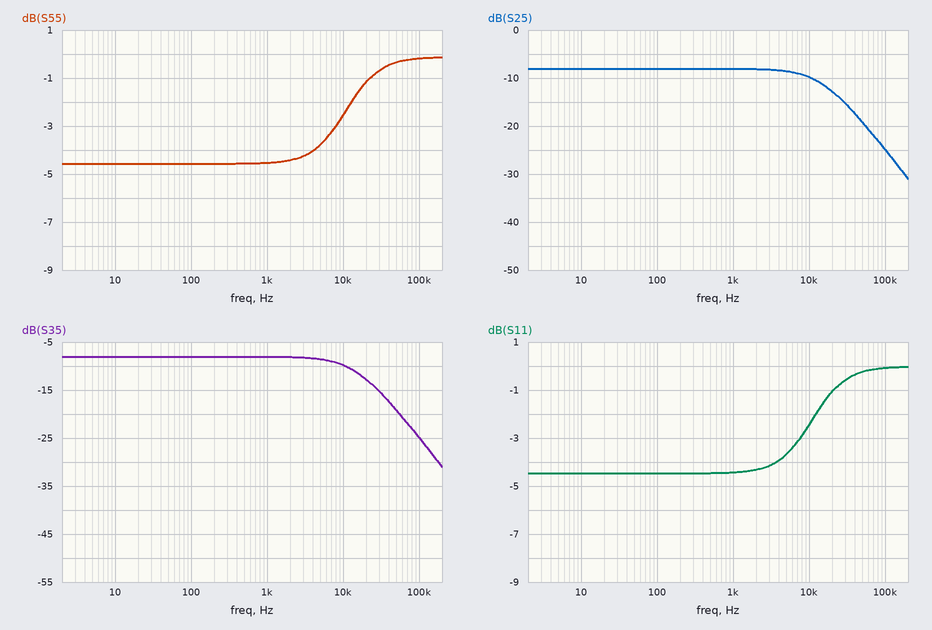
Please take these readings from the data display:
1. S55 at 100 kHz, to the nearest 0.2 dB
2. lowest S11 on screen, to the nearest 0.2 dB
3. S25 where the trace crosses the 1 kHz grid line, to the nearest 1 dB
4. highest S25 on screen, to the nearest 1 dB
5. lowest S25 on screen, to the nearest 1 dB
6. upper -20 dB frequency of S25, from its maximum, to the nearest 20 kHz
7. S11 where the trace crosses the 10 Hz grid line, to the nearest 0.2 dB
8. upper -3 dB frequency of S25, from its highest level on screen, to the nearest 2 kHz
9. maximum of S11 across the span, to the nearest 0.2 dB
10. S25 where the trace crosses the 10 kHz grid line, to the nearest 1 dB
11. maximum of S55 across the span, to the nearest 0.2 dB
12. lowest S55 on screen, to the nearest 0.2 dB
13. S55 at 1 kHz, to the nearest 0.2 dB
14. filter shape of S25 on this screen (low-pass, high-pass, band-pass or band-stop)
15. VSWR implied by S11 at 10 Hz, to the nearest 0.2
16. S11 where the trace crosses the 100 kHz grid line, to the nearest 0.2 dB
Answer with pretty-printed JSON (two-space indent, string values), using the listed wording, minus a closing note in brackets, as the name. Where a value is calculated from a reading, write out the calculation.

{
  "S55 at 100 kHz, to the nearest 0.2 dB": "-0.2 dB",
  "lowest S11 on screen, to the nearest 0.2 dB": "-4.4 dB",
  "S25 where the trace crosses the 1 kHz grid line, to the nearest 1 dB": "-8 dB",
  "highest S25 on screen, to the nearest 1 dB": "-8 dB",
  "lowest S25 on screen, to the nearest 1 dB": "-31 dB",
  "upper -20 dB frequency of S25, from its maximum, to the nearest 20 kHz": "140 kHz",
  "S11 where the trace crosses the 10 Hz grid line, to the nearest 0.2 dB": "-4.4 dB",
  "upper -3 dB frequency of S25, from its highest level on screen, to the nearest 2 kHz": "14 kHz",
  "maximum of S11 across the span, to the nearest 0.2 dB": "0.0 dB",
  "S25 where the trace crosses the 10 kHz grid line, to the nearest 1 dB": "-10 dB",
  "maximum of S55 across the span, to the nearest 0.2 dB": "-0.2 dB",
  "lowest S55 on screen, to the nearest 0.2 dB": "-4.6 dB",
  "S55 at 1 kHz, to the nearest 0.2 dB": "-4.6 dB",
  "filter shape of S25 on this screen": "low-pass",
  "VSWR implied by S11 at 10 Hz, to the nearest 0.2": "|Γ| = 10^(-4.4/20) = 0.6026; VSWR = (1 + 0.6026)/(1 − 0.6026) ≈ 4.0",
  "S11 where the trace crosses the 100 kHz grid line, to the nearest 0.2 dB": "0.0 dB"
}
